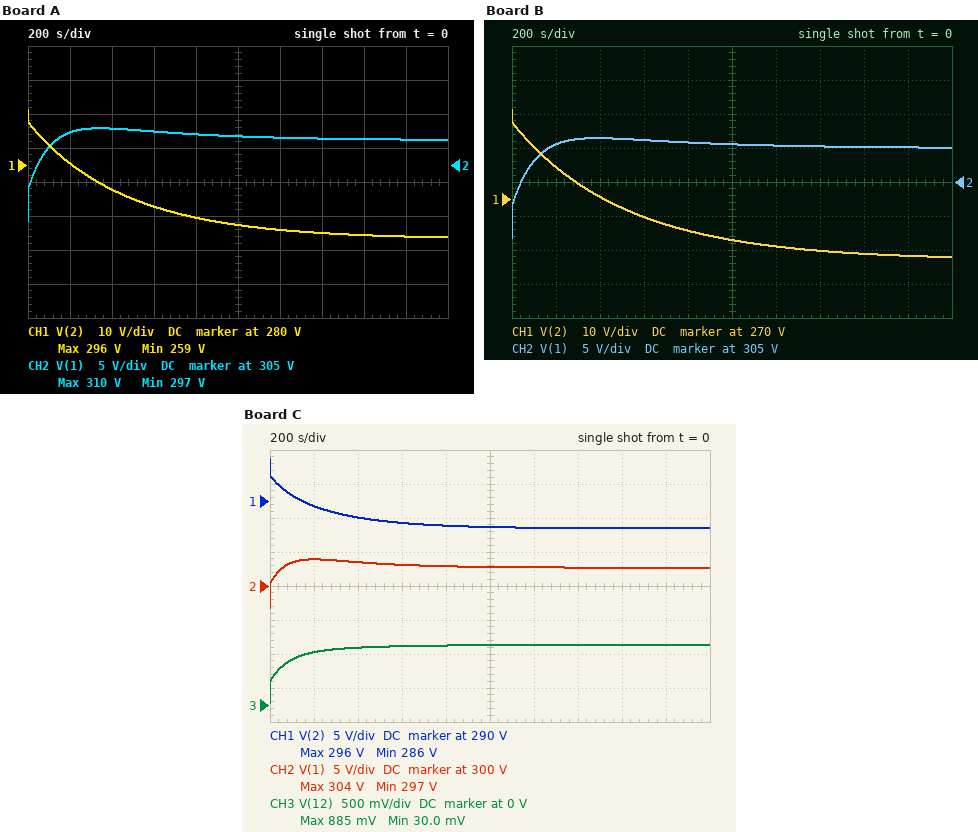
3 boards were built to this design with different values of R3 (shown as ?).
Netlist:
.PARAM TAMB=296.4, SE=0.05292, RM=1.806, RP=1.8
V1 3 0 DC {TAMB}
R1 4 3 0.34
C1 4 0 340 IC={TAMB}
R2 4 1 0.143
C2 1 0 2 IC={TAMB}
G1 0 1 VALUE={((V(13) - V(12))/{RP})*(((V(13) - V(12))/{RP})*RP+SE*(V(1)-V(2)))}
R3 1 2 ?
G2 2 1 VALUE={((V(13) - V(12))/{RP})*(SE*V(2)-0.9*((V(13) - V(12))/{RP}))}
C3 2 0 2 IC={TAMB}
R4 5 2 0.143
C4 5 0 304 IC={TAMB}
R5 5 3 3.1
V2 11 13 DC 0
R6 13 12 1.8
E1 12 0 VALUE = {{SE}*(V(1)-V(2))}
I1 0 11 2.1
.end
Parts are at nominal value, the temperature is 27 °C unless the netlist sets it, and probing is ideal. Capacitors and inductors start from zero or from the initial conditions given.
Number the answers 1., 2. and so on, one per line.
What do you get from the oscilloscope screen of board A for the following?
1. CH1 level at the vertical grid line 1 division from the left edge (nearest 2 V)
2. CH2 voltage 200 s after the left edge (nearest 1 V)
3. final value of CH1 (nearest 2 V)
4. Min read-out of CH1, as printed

1. 280 V
2. 310 V
3. 258 V
4. 259 V
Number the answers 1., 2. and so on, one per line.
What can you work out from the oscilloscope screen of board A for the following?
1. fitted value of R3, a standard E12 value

1. 3.9 Ω
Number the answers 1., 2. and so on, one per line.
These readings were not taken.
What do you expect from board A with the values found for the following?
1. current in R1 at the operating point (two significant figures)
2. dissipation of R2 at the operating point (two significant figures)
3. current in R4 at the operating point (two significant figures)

1. 25 A
2. 92 W
3. 12 A
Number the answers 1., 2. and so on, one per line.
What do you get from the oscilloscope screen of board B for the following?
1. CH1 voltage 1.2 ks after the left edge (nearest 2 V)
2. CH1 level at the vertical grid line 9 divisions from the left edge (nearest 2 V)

1. 256 V
2. 254 V
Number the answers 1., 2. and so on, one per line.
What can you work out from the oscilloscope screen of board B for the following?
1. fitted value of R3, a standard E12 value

1. 5.6 Ω
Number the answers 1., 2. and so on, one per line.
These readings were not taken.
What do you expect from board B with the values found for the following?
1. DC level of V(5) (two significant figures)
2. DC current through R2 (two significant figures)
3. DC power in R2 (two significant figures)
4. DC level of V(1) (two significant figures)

1. 250 V
2. 28 A
3. 110 W
4. 310 V
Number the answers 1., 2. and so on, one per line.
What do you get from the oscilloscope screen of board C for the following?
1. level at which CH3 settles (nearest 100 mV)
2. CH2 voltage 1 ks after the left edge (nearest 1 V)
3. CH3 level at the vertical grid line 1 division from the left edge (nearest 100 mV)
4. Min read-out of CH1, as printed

1. 900 mV
2. 303 V
3. 800 mV
4. 286 V
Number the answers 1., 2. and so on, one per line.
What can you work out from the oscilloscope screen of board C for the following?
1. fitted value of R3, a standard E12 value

1. 0.68 Ω
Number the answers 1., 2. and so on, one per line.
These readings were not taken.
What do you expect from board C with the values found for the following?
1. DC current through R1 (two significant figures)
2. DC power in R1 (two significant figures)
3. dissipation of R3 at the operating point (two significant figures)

1. 13 A
2. 58 W
3. 410 W
